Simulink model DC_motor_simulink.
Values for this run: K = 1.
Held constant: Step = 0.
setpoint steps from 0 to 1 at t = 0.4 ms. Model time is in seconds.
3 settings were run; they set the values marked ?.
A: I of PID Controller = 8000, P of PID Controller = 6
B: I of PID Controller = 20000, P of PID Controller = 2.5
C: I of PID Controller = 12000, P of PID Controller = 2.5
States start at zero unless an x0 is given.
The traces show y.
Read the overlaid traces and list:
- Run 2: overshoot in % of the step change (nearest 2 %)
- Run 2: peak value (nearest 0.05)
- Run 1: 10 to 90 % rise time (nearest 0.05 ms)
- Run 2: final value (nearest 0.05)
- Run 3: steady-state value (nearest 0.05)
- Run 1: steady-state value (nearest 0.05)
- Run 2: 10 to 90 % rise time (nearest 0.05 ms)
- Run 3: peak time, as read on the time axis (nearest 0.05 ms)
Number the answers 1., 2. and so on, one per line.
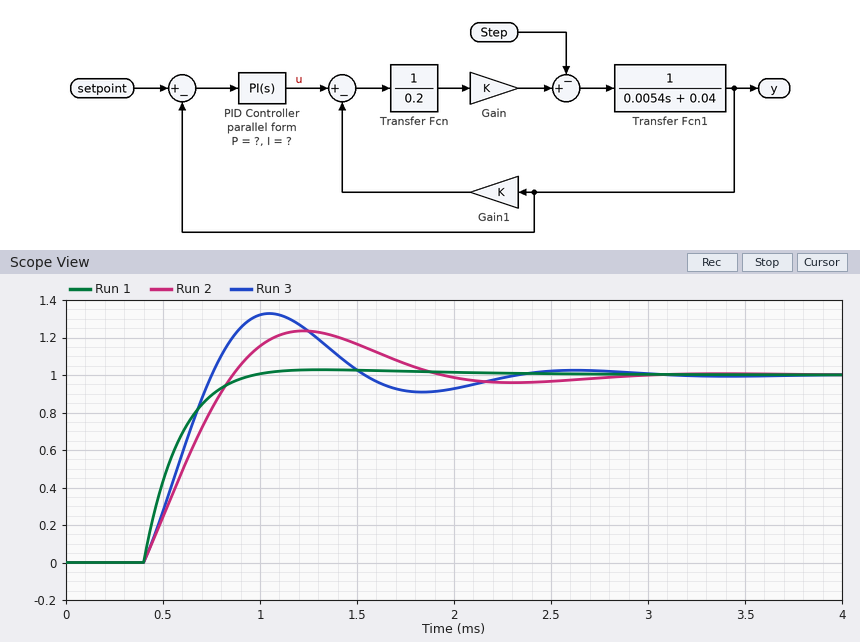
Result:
1. 24 %
2. 1.25
3. 0.35 ms
4. 1.00
5. 1.00
6. 1.00
7. 0.35 ms
8. 1.05 ms
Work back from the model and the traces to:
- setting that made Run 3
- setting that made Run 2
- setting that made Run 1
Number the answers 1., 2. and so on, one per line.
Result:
1. B
2. C
3. A
